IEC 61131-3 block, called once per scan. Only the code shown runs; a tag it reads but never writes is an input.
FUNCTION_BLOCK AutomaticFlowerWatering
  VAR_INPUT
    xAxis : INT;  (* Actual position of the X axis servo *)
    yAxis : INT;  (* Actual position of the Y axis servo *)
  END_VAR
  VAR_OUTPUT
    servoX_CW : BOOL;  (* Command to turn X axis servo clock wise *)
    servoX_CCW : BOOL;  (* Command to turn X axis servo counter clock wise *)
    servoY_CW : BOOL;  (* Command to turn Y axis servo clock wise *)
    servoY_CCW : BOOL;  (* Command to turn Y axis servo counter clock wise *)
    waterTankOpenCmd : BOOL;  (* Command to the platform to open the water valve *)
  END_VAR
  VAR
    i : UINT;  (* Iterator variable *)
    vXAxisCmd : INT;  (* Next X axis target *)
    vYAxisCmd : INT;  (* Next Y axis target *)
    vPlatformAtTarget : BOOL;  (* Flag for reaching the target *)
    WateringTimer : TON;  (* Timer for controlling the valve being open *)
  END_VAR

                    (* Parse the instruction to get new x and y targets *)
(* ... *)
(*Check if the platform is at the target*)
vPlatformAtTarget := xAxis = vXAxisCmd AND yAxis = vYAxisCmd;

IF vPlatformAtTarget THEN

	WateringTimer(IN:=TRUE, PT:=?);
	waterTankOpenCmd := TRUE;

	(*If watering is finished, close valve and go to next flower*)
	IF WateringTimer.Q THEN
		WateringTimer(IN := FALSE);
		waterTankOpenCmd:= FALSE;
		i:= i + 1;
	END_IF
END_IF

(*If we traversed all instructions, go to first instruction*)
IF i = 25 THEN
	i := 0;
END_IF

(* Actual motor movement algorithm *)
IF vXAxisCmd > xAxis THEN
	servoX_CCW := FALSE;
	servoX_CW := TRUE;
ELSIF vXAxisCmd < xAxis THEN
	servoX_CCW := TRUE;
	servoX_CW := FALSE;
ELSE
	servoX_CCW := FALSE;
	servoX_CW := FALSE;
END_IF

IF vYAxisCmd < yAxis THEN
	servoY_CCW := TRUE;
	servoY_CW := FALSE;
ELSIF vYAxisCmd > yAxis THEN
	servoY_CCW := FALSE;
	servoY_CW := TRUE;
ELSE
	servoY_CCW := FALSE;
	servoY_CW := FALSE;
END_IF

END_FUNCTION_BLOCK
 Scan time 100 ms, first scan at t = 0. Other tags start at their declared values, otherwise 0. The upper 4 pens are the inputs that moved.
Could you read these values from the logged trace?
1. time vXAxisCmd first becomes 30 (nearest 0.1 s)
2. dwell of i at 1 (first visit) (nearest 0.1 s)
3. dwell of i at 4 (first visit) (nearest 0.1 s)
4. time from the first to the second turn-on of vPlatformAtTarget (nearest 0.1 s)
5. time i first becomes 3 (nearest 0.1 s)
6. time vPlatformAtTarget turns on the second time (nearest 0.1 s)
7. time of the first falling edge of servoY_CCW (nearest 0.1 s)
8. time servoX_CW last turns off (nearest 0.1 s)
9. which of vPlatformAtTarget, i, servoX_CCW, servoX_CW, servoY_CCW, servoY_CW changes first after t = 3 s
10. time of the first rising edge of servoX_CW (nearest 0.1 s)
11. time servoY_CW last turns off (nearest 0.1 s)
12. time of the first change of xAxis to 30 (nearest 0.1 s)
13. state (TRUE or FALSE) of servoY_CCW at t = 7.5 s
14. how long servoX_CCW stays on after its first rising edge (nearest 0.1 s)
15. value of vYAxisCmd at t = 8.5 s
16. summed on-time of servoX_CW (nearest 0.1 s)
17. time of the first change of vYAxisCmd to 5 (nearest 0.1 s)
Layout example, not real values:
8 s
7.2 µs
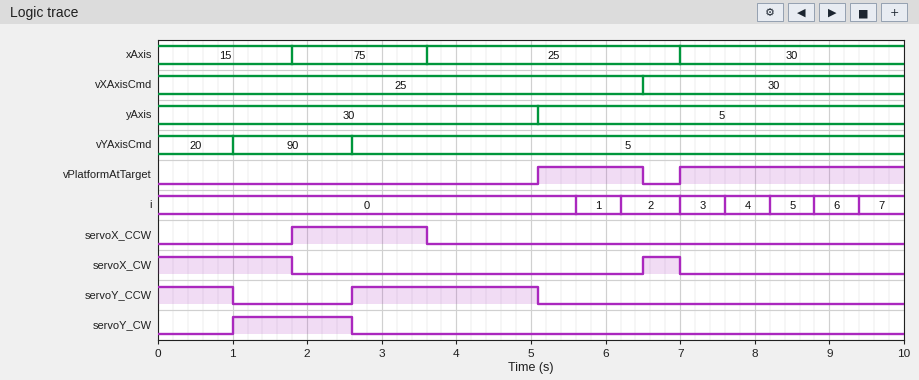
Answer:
6.5 s
0.6 s
0.6 s
1.9 s
7.0 s
7.0 s
1.0 s
7.0 s
servoX_CCW
6.5 s
2.6 s
7.0 s
FALSE
1.8 s
5
2.3 s
2.6 s
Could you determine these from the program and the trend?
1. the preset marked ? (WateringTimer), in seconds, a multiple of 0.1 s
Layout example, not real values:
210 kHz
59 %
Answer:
0.5 s
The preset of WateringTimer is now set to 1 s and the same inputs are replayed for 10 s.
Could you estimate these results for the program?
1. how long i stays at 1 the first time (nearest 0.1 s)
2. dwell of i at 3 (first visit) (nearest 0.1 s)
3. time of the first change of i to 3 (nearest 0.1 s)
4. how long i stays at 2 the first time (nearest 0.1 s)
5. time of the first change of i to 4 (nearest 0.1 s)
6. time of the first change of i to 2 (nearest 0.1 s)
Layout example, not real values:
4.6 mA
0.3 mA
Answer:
1.1 s
1.1 s
8.3 s
1.1 s
9.4 s
7.2 s
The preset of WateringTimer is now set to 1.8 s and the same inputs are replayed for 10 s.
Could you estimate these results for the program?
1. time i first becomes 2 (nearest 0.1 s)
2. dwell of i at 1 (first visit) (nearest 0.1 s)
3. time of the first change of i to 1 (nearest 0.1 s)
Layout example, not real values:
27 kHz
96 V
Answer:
8.9 s
1.9 s
7.0 s
